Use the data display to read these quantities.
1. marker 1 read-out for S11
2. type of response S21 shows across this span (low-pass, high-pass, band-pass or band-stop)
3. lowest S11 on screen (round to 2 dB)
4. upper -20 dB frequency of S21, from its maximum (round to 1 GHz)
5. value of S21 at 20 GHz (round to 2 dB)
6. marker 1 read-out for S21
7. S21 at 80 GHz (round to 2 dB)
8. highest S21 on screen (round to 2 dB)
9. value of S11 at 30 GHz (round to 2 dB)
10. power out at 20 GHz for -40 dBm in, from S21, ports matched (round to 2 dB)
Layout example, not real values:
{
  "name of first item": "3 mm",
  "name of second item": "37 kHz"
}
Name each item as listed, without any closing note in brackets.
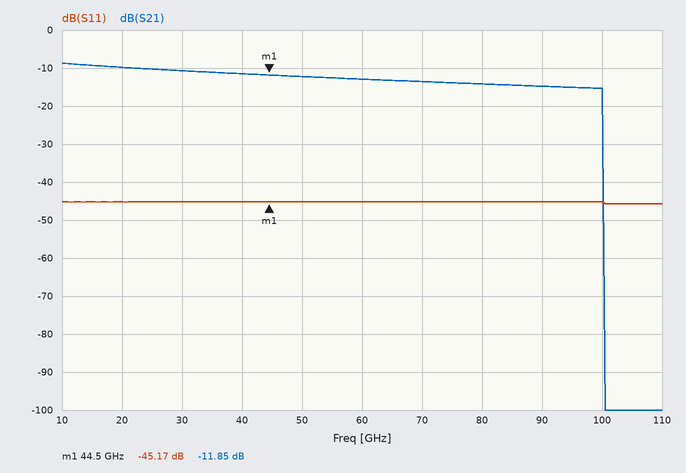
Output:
{
  "marker 1 read-out for S11": "-45.17 dB",
  "type of response S21 shows across this span": "low-pass",
  "lowest S11 on screen": "-46 dB",
  "upper -20 dB frequency of S21, from its maximum": "100 GHz",
  "value of S21 at 20 GHz": "-10 dB",
  "marker 1 read-out for S21": "-11.85 dB",
  "S21 at 80 GHz": "-14 dB",
  "highest S21 on screen": "-8 dB",
  "value of S11 at 30 GHz": "-46 dB",
  "power out at 20 GHz for -40 dBm in, from S21, ports matched": "-50 dBm"
}
